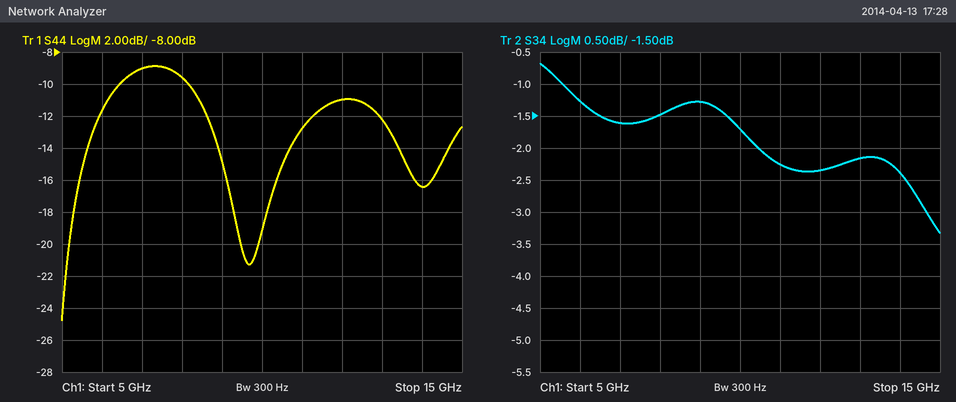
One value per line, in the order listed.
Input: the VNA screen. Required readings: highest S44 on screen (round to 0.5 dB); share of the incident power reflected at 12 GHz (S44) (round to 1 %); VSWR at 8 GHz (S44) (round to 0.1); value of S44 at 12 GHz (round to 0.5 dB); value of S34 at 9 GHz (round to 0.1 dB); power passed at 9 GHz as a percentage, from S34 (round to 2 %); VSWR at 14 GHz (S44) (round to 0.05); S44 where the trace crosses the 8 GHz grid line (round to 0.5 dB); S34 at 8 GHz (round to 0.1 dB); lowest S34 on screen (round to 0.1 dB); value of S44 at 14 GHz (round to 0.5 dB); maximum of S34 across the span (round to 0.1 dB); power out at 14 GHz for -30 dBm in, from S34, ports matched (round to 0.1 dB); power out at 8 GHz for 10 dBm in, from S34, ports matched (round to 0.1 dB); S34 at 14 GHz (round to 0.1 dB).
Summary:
-9.0 dB
8 %
2.0
-11.0 dB
-1.3 dB
74 %
1.35
-9.5 dB
-1.5 dB
-3.3 dB
-16.5 dB
-0.7 dB
-32.4 dBm
8.5 dBm
-2.4 dB
